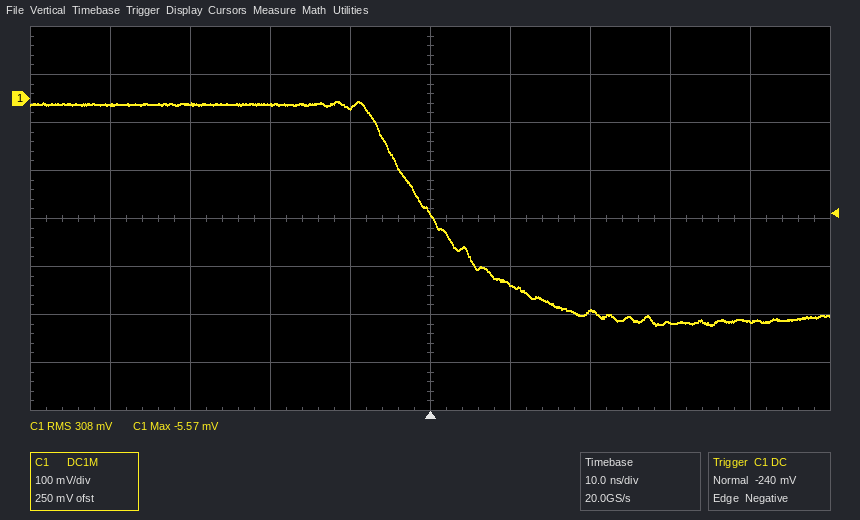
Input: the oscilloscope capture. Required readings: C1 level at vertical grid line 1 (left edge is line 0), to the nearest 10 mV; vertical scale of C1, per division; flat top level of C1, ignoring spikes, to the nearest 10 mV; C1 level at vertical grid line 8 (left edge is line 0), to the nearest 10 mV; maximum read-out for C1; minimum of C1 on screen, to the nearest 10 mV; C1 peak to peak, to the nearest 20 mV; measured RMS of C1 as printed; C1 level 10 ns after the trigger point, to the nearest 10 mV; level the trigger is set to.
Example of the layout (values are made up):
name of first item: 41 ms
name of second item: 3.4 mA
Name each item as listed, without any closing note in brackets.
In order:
C1 level at vertical grid line 1 (left edge is line 0), to the nearest 10 mV: -10 mV
vertical scale of C1, per division: 100 mV
flat top level of C1, ignoring spikes, to the nearest 10 mV: -10 mV
C1 level at vertical grid line 8 (left edge is line 0), to the nearest 10 mV: -470 mV
maximum read-out for C1: -5.57 mV
minimum of C1 on screen, to the nearest 10 mV: -470 mV
C1 peak to peak, to the nearest 20 mV: 460 mV
measured RMS of C1 as printed: 308 mV
C1 level 10 ns after the trigger point, to the nearest 10 mV: -390 mV
level the trigger is set to: -240 mV
